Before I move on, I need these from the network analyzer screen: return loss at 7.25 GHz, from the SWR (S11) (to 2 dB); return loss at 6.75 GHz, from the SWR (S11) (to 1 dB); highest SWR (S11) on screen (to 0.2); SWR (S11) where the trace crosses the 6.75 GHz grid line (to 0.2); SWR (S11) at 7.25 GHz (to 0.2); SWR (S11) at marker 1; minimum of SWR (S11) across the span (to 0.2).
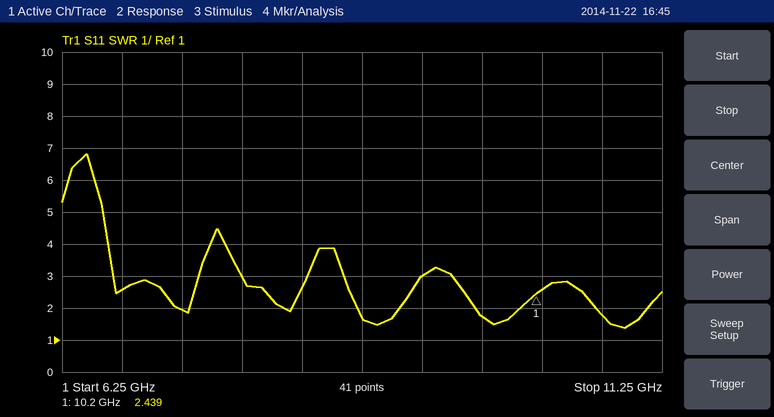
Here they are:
10 dB
7 dB
6.8
2.6
2.0
2.439
1.4
